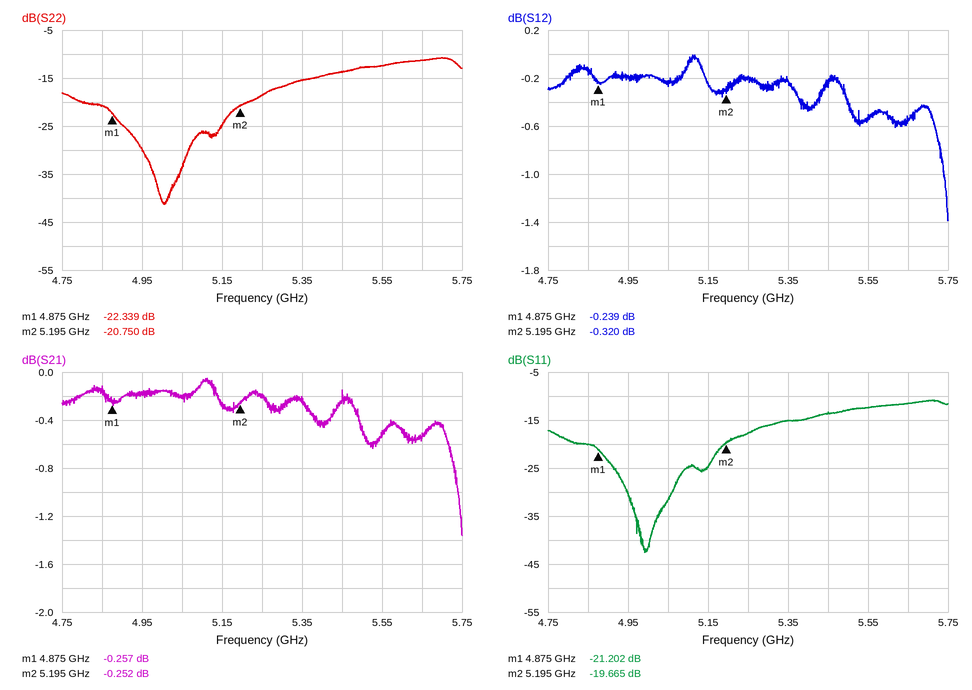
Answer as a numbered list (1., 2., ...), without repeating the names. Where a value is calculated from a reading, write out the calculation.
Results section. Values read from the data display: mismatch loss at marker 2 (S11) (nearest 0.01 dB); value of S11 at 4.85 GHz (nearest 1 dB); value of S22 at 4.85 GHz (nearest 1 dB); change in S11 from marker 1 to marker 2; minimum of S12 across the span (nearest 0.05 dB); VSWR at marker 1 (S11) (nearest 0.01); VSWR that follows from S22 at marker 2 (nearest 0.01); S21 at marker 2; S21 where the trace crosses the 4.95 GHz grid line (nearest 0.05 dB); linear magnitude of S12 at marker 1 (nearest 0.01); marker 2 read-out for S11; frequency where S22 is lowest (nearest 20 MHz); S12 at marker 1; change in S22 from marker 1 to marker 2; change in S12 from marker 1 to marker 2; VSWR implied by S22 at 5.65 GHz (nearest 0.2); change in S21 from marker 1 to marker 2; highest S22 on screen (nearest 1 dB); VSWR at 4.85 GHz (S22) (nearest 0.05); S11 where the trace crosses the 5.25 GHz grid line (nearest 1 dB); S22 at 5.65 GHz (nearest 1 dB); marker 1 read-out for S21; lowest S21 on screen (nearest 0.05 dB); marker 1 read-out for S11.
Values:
1. −10 log10(1 − 10^(-19.665/10)) ≈ 0.05 dB
2. -20 dB
3. -21 dB
4. -19.665 − (-21.202) = 1.537 dB
5. -1.40 dB
6. (1 + 0.0871)/(1 − 0.0871) ≈ 1.19
7. (1 + 0.0917)/(1 − 0.0917) ≈ 1.20
8. -0.252 dB
9. -0.15 dB
10. 10^(-0.239/20) ≈ 0.97
11. -19.665 dB
12. 5.00 GHz
13. -0.239 dB
14. -20.75 − (-22.339) = 1.589 dB
15. -0.32 − (-0.239) = -0.081 dB
16. |Γ| = 10^(-11/20) = 0.2818; VSWR = (1 + 0.2818)/(1 − 0.2818) ≈ 1.8
17. -0.252 − (-0.257) = 0.005 dB
18. -11 dB
19. |Γ| = 10^(-21/20) = 0.0891; VSWR = (1 + 0.0891)/(1 − 0.0891) ≈ 1.20
20. -18 dB
21. -11 dB
22. -0.257 dB
23. -1.35 dB
24. -21.202 dB
